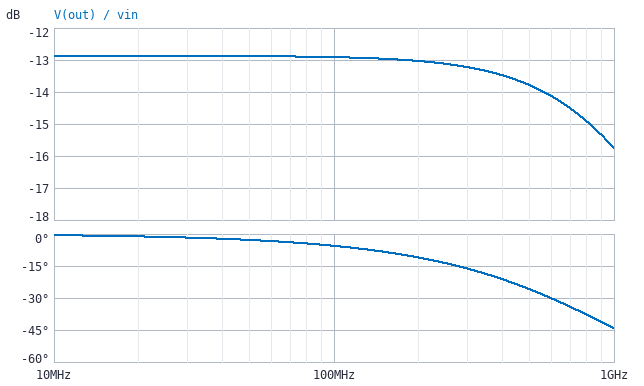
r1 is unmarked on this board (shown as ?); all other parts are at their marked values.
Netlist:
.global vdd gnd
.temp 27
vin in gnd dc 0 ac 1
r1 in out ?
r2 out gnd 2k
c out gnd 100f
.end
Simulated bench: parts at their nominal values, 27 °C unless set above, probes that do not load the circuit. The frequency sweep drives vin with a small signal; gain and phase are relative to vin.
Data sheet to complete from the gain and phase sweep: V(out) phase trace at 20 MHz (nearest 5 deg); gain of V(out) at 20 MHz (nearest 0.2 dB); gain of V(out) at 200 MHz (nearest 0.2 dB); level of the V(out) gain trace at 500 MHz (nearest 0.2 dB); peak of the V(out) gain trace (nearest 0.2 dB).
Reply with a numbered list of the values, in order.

1. 0 deg
2. -12.8 dB
3. -13.0 dB
4. -13.8 dB
5. -12.8 dB
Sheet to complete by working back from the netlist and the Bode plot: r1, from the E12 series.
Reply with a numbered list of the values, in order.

1. 6.8 kΩ
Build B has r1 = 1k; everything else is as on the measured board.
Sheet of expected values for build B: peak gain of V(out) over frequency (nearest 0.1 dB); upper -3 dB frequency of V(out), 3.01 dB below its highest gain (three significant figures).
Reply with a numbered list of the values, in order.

1. -3.5 dB
2. 2.39 GHz
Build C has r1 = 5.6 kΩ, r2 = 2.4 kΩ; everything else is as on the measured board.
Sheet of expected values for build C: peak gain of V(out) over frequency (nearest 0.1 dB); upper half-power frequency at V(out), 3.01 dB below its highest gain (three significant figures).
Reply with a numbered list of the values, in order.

1. -10.5 dB
2. 947 MHz
